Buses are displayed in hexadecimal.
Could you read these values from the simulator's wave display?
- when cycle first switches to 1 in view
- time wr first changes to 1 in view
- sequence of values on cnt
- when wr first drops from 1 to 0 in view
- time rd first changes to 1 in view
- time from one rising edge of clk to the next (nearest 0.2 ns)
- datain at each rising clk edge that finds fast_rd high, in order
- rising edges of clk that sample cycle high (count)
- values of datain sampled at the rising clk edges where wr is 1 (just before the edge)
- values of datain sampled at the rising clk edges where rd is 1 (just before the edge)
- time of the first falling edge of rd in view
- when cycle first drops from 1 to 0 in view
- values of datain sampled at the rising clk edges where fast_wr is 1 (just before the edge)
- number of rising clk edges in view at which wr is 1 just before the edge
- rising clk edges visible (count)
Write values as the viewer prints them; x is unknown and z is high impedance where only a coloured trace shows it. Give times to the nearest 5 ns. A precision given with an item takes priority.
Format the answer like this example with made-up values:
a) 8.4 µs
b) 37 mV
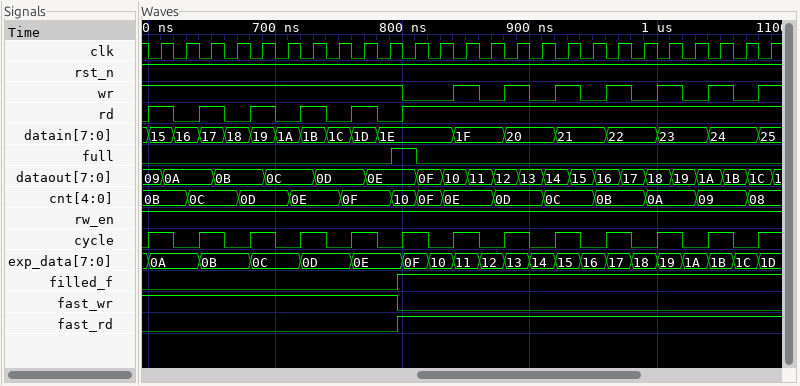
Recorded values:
a) 600 ns
b) 840 ns
c) 0B, 0C, 0D, 0E, 0F, 10, 0F, 0E, 0D, 0C, 0B, 0A, 09, 08
d) 800 ns
e) 600 ns
f) 20 ns
g) 1E, 1E, 1F, 1F, 20, 20, 21, 21, 22, 22, 23, 23, 24, 24, 25
h) 13
i) 15, 16, 17, 18, 19, 1A, 1B, 1C, 1D, 1E, 1F, 20, 21, 22, 23, 24, 25
j) 15, 17, 19, 1B, 1D, 1E, 1E, 1F, 1F, 20, 20, 21, 21, 22, 22, 23, 23, 24, 24, 25
k) 620 ns
l) 620 ns
m) 15, 16, 17, 18, 19, 1A, 1B, 1C, 1D, 1E
n) 17
o) 25
